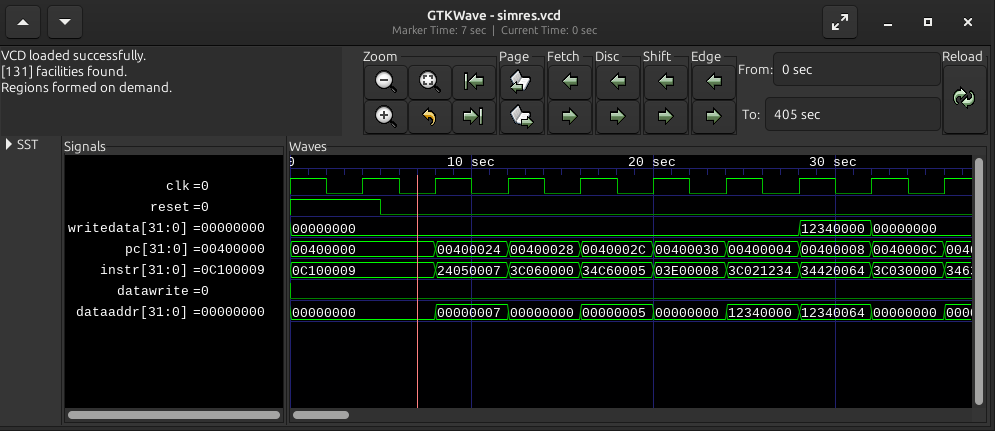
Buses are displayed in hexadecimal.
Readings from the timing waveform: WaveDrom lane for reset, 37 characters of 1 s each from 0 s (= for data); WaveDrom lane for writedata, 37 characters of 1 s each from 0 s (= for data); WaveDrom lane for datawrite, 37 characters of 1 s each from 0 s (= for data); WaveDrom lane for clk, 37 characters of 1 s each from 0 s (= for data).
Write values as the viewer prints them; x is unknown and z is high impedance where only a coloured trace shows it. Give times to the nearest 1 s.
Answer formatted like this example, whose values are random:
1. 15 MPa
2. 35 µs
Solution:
1. {name: 'reset', wave: '1....0...............................'}
2. {name: 'writedata', wave: '=...........................=...=....', data: '00000000 12340000 00000000'}
3. {name: 'datawrite', wave: '0....................................'}
4. {name: 'clk', wave: '1.0.1.0.1.0.1.0.1.0.1.0.1.0.1.0.1.0.1'}
